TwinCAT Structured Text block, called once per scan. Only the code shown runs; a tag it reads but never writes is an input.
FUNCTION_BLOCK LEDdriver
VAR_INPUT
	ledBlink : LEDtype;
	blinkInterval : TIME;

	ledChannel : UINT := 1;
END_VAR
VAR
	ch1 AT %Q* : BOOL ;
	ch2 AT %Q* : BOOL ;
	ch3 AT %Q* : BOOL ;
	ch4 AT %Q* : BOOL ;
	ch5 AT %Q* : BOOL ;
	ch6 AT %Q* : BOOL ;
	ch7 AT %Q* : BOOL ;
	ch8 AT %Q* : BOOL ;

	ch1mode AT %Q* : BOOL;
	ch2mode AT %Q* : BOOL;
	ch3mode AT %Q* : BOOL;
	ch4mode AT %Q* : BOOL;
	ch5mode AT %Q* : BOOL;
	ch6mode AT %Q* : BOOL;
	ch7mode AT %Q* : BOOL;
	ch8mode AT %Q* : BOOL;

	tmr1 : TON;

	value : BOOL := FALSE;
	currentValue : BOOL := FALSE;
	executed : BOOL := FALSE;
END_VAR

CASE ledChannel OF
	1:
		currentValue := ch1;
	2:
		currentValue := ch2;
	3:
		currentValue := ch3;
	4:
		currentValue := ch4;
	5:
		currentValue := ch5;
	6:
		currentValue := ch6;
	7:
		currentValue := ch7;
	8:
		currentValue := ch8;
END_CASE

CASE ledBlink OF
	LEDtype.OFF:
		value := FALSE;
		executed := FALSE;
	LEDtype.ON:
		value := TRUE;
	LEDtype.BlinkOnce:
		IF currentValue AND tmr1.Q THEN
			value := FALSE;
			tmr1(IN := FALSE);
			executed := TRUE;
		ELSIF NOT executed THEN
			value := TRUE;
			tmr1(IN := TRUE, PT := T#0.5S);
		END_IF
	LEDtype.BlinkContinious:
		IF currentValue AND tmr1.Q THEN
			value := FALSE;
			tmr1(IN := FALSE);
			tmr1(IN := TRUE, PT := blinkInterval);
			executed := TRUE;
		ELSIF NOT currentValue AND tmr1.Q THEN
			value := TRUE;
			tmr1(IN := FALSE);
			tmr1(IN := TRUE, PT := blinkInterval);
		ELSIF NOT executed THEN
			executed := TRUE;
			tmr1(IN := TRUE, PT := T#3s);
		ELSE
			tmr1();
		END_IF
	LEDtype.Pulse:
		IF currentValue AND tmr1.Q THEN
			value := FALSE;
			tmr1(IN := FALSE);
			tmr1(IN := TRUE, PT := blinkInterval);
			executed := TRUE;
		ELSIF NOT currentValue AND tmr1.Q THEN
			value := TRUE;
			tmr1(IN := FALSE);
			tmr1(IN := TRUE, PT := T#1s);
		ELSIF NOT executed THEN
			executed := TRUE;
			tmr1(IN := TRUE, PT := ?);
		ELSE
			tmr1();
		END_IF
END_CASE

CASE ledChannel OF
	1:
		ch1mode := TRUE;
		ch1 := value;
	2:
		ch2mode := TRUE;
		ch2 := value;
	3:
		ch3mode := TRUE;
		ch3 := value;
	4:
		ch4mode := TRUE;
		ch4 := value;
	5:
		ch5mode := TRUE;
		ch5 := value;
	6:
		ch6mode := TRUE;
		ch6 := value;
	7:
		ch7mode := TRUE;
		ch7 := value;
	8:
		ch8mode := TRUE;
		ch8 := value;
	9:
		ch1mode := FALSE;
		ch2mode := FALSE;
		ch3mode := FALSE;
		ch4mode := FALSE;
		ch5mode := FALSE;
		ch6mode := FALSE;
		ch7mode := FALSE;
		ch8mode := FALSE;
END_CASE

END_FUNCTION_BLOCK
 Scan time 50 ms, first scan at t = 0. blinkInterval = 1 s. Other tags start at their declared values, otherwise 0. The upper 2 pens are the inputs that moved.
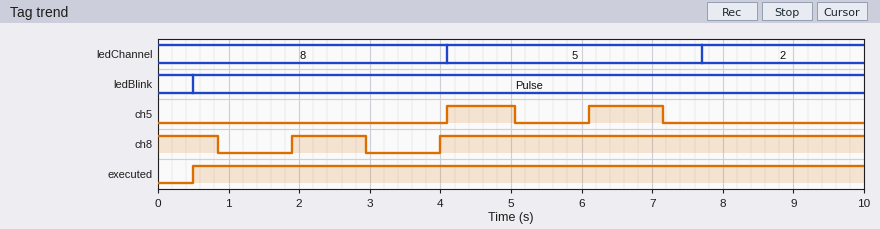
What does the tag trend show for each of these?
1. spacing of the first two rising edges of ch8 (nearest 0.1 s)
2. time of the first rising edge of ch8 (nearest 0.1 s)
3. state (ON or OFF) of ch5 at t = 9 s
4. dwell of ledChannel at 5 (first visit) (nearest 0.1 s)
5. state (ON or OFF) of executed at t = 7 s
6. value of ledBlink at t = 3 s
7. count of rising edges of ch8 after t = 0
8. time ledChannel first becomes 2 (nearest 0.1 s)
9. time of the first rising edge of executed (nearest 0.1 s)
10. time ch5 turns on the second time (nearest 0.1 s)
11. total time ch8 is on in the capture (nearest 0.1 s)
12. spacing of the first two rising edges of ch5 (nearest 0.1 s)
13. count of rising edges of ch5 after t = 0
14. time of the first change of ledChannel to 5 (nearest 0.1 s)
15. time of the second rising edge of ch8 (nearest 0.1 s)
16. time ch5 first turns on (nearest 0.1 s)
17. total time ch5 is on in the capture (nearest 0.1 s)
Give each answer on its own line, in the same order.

2.1 s
1.9 s
OFF
3.6 s
ON
Pulse
2
7.7 s
0.5 s
6.1 s
7.9 s
2.0 s
2
4.1 s
4.0 s
4.1 s
2.0 s
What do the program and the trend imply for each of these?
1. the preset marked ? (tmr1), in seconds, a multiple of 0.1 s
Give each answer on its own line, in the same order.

0.8 s
